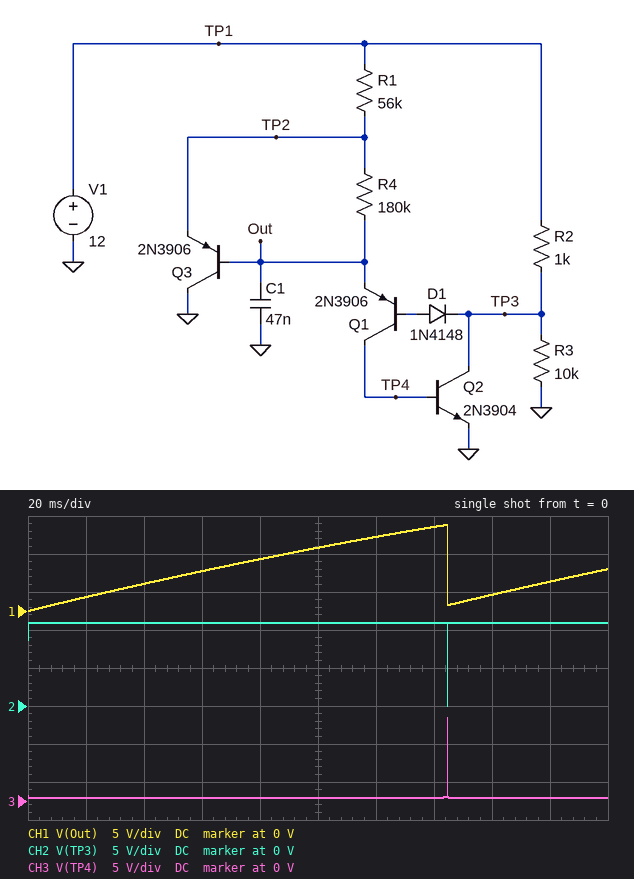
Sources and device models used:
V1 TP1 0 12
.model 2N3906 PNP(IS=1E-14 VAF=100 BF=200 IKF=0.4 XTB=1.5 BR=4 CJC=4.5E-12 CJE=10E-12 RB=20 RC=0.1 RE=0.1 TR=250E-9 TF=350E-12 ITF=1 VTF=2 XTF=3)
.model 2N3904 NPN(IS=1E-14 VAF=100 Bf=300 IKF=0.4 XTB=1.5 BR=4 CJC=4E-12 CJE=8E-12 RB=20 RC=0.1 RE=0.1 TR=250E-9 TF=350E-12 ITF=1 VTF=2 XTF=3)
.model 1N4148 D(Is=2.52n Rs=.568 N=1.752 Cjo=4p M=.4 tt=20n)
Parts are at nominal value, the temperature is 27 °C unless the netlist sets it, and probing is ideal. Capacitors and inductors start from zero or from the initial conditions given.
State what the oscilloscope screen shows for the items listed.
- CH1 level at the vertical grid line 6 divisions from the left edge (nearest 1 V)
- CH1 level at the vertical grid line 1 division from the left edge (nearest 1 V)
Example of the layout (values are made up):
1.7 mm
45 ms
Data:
10 V
2 V
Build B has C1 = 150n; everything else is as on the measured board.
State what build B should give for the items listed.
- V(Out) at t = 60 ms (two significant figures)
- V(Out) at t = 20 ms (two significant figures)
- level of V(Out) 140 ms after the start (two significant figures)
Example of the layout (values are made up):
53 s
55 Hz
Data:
1.7 V
580 mV
3.9 V
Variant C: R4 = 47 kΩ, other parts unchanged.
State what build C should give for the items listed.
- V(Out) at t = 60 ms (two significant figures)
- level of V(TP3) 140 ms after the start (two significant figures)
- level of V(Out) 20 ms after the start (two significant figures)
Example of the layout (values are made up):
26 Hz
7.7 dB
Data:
5.8 V
11 V
5.7 V
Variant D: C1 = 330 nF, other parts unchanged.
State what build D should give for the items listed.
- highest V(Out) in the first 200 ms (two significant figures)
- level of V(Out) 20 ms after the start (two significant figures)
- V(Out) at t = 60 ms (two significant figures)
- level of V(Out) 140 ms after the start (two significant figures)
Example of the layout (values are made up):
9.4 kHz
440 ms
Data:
2.6 V
270 mV
790 mV
1.8 V
